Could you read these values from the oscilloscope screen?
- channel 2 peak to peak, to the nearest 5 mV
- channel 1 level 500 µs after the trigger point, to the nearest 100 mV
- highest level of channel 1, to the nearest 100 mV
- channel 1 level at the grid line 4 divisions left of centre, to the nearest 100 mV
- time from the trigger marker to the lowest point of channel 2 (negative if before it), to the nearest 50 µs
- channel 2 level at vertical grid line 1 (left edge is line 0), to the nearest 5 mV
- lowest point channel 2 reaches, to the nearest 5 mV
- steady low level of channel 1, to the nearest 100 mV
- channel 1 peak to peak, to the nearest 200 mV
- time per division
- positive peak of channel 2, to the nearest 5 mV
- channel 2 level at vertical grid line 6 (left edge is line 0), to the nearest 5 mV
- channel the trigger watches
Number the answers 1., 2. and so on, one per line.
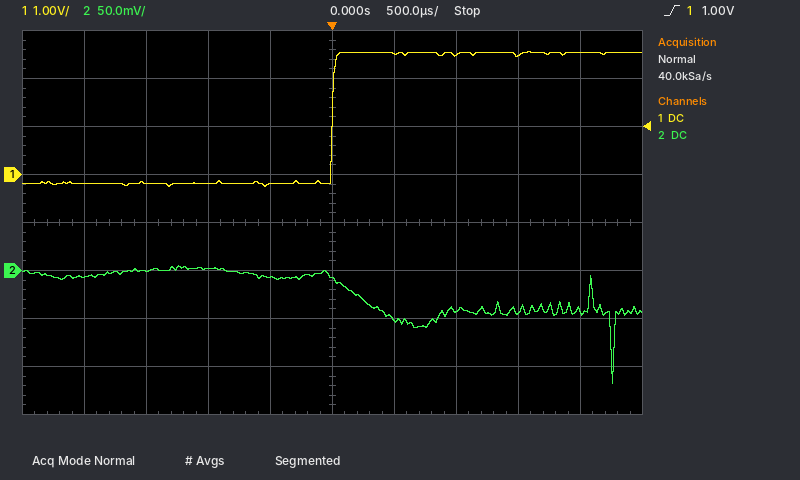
1. 125 mV
2. 2.5 V
3. 2.6 V
4. -200 mV
5. +2.25 ms
6. -5 mV
7. -120 mV
8. -200 mV
9. 2.8 V
10. 500 µs
11. 5 mV
12. -50 mV
13. channel 1
